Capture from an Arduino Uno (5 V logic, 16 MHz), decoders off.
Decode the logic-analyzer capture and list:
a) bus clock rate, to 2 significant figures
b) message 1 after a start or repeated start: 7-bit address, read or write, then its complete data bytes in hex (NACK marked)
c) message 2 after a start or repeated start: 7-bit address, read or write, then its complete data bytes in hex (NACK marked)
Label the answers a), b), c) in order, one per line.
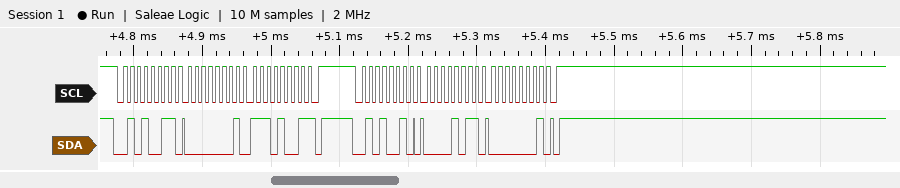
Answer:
a) 100 kHz
b) 0x29 read: 01 E9 NACK
c) 0x29 write: 0B 01
